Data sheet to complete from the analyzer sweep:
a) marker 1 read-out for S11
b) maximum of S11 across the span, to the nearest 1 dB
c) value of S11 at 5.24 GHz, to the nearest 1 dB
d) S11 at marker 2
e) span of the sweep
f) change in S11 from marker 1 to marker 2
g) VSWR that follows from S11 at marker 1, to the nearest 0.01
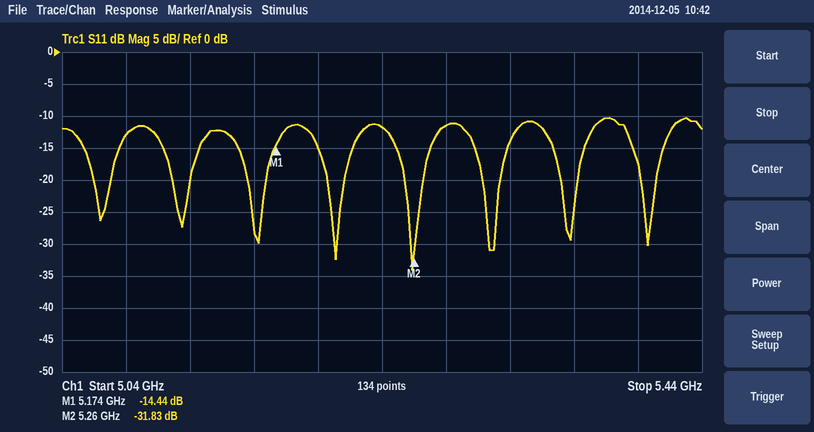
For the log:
-14.44 dB
-10 dB
-12 dB
-31.83 dB
400 MHz
-17.39 dB
1.47
